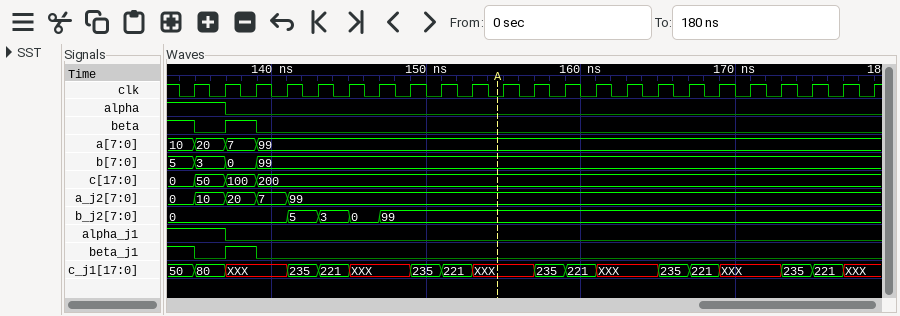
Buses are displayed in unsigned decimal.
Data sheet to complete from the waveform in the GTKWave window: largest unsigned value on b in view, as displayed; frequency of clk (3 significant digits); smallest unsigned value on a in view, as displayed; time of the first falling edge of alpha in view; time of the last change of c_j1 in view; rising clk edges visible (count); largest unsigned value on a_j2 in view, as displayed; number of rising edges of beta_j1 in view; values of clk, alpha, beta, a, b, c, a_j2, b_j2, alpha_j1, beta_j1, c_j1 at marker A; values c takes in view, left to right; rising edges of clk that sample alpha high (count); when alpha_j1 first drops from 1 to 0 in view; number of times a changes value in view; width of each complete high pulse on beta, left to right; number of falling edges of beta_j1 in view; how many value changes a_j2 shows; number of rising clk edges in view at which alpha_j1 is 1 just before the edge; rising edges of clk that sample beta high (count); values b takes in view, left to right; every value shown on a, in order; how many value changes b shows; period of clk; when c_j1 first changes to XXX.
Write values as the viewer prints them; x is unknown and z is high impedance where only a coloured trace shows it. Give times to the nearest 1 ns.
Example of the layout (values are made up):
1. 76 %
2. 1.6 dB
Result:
1. 99
2. 500 MHz
3. 7
4. 137 ns
5. 177 ns
6. 23
7. 99
8. 1
9. clk=0, alpha=0, beta=0, a=99, b=99, c=200, a_j2=99, b_j2=99, alpha_j1=0, beta_j1=0, c_j1=XXX
10. 0, 50, 100, 200
11. 2
12. 137 ns
13. 3
14. 2 ns
15. 2
16. 4
17. 2
18. 2
19. 5, 3, 0, 99
20. 10, 20, 7, 99
21. 3
22. 2 ns
23. 137 ns
